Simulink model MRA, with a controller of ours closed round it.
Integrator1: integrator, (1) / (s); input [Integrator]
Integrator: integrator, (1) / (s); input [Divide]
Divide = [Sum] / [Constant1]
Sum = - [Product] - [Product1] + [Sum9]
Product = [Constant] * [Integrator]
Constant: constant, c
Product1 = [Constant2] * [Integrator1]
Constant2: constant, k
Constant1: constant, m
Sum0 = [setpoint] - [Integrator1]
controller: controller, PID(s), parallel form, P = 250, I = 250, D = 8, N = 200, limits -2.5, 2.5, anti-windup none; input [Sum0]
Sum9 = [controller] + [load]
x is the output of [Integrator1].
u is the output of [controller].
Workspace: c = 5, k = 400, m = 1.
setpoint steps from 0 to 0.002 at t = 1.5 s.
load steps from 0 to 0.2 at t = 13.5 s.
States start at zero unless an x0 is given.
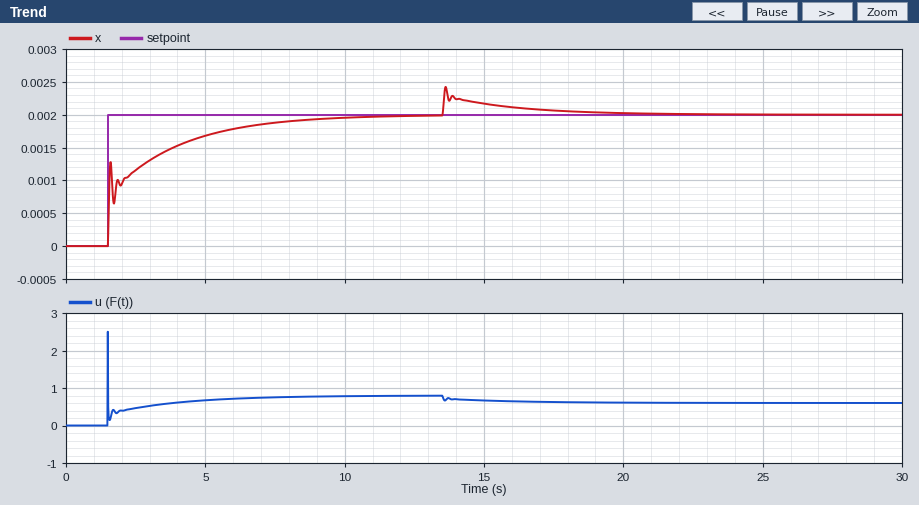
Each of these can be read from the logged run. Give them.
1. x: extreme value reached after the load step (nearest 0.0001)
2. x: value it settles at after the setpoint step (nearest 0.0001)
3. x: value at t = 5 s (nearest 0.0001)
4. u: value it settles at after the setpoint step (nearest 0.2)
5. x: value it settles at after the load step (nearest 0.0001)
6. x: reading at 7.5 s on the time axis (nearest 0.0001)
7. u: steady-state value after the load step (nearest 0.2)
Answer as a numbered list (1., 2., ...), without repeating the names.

1. 0.0024
2. 0.0020
3. 0.0017
4. 0.8
5. 0.0020
6. 0.0019
7. 0.6
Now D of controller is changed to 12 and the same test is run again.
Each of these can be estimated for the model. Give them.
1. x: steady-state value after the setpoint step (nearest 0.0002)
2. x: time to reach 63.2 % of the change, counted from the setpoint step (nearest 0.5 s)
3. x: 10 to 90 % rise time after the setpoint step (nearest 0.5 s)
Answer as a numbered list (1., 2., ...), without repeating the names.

1. 0.0020
2. 1.5 s
3. 4.5 s
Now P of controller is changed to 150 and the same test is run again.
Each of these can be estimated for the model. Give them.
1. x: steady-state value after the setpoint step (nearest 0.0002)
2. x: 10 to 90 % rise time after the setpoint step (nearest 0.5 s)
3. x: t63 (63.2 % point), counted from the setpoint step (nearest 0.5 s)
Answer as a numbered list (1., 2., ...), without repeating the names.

1. 0.0020
2. 4.5 s
3. 1.5 s
